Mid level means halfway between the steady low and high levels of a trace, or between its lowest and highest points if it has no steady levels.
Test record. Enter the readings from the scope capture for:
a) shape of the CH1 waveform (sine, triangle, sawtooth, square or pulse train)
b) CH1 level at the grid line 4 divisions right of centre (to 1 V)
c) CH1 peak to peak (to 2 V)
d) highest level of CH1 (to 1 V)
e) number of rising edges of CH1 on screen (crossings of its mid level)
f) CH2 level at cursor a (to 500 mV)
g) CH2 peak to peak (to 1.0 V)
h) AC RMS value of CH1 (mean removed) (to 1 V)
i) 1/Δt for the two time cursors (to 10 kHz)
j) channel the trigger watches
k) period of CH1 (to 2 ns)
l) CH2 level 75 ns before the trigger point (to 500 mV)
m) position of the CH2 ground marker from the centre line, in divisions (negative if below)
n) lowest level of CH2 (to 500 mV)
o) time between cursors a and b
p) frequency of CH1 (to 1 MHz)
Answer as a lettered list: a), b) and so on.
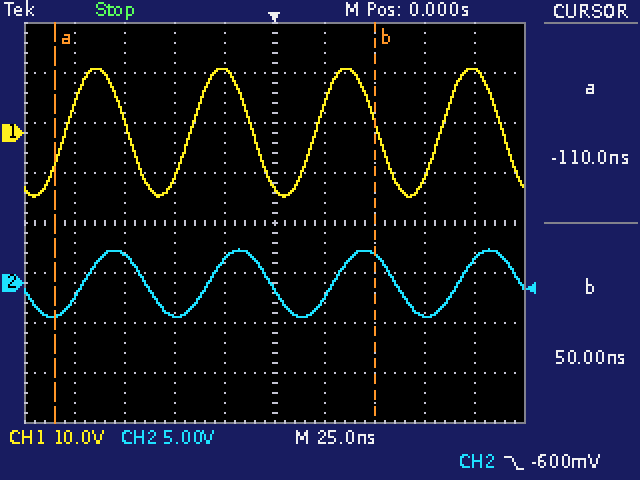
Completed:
a) sine
b) 13 V
c) 26 V
d) 13 V
e) 4
f) -3.0 V
g) 7.0 V
h) 9 V
i) 6.25 MHz
j) CH2
k) 62 ns
l) 3.0 V
m) -1.2 div
n) -3.5 V
o) 160.0 ns
p) 16 MHz
